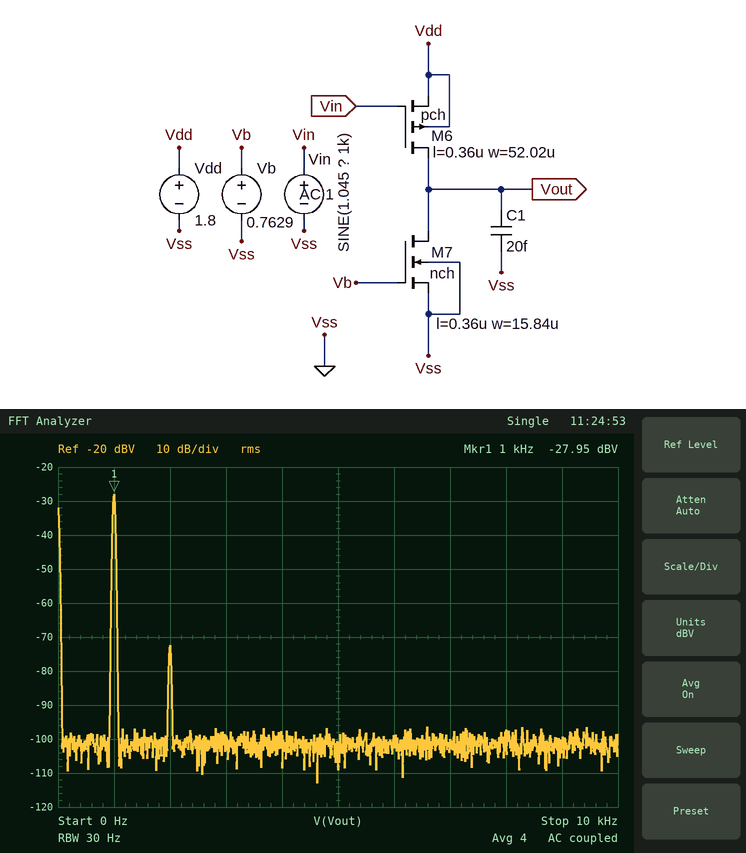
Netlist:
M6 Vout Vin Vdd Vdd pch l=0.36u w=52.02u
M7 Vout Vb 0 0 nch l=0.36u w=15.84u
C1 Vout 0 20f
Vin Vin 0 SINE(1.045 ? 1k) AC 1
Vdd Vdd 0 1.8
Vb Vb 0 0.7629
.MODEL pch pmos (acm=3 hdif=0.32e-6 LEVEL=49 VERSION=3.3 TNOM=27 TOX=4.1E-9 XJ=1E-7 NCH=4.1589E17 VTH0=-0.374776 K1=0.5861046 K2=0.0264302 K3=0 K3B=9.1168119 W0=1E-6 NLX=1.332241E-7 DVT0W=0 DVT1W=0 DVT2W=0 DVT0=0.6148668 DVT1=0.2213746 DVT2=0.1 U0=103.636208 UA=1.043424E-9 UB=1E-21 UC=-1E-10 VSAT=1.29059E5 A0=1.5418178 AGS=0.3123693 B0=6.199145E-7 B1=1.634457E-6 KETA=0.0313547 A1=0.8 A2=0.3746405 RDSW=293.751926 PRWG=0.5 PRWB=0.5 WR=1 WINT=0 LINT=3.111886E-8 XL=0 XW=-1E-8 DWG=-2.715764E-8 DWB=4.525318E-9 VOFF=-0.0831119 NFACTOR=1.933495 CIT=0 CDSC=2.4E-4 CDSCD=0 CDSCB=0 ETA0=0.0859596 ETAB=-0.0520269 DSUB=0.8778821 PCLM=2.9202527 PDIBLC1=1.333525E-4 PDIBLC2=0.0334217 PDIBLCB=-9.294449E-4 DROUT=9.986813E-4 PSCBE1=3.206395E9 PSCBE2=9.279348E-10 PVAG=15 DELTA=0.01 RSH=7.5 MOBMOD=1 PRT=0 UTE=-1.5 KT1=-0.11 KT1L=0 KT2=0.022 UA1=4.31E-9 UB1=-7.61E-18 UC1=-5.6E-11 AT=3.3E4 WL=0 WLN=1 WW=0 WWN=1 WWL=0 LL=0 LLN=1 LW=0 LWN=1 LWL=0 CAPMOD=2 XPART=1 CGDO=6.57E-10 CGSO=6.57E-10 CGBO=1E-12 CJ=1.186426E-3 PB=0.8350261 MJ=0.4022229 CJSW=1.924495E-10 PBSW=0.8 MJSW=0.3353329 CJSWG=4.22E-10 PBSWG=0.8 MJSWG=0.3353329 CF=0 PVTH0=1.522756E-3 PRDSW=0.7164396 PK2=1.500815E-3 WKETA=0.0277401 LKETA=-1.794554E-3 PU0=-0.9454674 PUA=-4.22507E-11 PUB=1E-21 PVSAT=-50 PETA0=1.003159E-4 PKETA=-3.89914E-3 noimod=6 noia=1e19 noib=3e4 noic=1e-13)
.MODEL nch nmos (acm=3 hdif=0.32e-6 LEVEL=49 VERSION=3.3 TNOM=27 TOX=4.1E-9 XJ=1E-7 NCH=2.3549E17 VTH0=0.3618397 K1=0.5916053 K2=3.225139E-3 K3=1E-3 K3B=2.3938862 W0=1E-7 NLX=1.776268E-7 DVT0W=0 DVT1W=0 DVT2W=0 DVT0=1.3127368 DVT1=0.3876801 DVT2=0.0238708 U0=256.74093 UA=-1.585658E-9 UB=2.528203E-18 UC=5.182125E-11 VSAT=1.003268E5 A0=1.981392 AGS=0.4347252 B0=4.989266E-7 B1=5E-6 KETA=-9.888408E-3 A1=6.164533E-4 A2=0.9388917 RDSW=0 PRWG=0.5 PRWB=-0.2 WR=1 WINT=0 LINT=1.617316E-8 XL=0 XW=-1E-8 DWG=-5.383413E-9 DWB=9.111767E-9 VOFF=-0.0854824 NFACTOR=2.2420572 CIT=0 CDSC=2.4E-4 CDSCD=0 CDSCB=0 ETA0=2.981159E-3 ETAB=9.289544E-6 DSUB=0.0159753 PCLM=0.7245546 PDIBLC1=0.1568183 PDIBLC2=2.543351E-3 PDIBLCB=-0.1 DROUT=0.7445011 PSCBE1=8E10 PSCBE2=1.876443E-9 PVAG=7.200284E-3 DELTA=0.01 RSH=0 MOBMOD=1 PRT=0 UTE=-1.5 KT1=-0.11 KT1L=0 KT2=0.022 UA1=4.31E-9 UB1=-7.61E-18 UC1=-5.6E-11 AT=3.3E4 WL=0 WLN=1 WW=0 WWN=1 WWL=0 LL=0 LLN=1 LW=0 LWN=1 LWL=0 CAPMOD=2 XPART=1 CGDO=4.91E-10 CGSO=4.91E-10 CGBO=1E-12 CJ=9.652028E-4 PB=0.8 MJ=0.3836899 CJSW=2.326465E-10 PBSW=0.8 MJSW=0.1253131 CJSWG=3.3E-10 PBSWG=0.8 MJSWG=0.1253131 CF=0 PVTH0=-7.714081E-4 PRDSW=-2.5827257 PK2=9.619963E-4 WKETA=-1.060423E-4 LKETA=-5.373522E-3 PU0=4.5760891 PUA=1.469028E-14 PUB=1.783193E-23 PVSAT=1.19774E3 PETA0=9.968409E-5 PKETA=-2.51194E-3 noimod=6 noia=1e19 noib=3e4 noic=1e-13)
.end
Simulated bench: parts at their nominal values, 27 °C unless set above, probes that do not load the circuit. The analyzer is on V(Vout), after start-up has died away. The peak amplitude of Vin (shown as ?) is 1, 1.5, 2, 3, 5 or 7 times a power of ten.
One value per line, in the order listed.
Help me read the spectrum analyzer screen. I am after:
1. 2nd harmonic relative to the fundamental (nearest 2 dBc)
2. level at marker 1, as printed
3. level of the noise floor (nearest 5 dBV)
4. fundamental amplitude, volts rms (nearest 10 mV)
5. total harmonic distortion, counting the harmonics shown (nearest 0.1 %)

-44 dBc
-27.95 dBV
-100 dBV
40 mV
0.6 %
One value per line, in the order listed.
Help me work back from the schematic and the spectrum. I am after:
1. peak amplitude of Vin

2 mV
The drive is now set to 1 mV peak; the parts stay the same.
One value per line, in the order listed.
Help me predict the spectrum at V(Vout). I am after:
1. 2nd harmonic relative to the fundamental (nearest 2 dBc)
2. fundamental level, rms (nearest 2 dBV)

-50 dBc
-34 dBV
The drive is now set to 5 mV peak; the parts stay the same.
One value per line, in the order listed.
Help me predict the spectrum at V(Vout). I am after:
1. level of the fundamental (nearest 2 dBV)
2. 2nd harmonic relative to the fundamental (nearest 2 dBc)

-20 dBV
-36 dBc
